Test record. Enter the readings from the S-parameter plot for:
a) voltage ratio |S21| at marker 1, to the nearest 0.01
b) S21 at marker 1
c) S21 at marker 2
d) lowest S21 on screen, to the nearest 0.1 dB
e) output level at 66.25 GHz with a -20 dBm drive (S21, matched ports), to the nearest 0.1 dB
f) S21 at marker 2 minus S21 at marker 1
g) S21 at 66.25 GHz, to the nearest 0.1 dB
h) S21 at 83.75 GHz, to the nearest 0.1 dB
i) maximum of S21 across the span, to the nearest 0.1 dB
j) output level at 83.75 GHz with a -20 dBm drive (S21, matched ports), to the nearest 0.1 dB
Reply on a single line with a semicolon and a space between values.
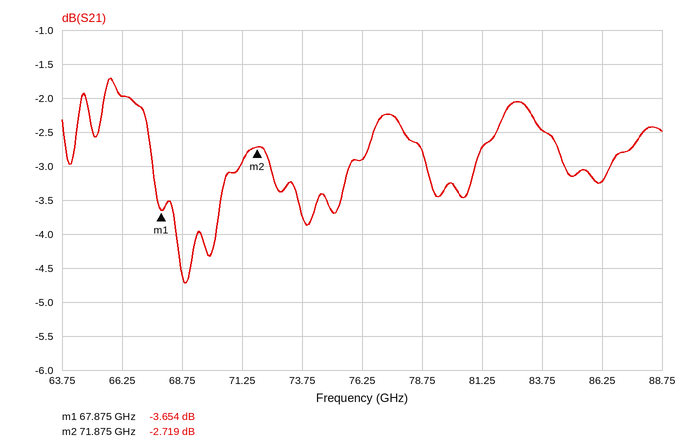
0.66; -3.654 dB; -2.719 dB; -4.7 dB; -22.0 dBm; 0.935 dB; -2.0 dB; -2.5 dB; -1.7 dB; -22.5 dBm
